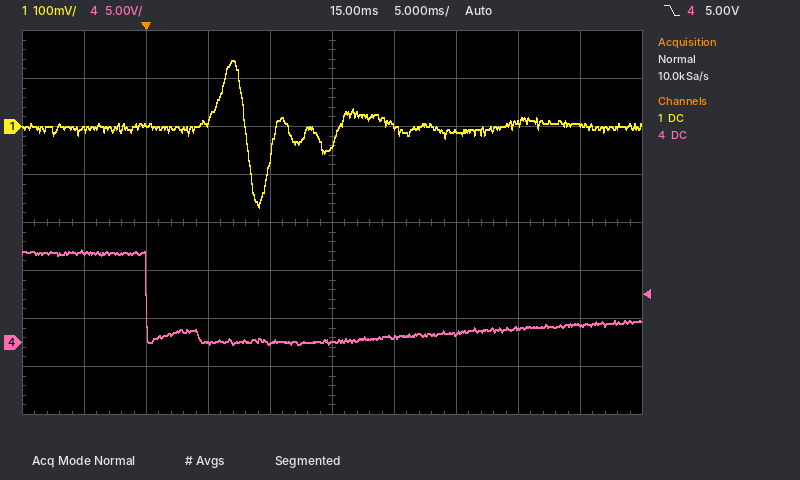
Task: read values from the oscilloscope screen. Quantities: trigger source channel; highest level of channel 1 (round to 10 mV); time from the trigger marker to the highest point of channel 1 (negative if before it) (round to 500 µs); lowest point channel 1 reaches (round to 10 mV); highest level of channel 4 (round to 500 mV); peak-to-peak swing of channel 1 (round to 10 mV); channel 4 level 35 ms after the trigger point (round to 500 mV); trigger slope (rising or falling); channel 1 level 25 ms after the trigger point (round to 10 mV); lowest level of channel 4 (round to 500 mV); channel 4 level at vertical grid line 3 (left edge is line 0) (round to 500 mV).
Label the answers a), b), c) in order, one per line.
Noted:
a) channel 4
b) 140 mV
c) +7.0 ms
d) -170 mV
e) 9.5 V
f) 310 mV
g) 2.0 V
h) falling
i) -10 mV
j) 0.0 V
k) 0.0 V
